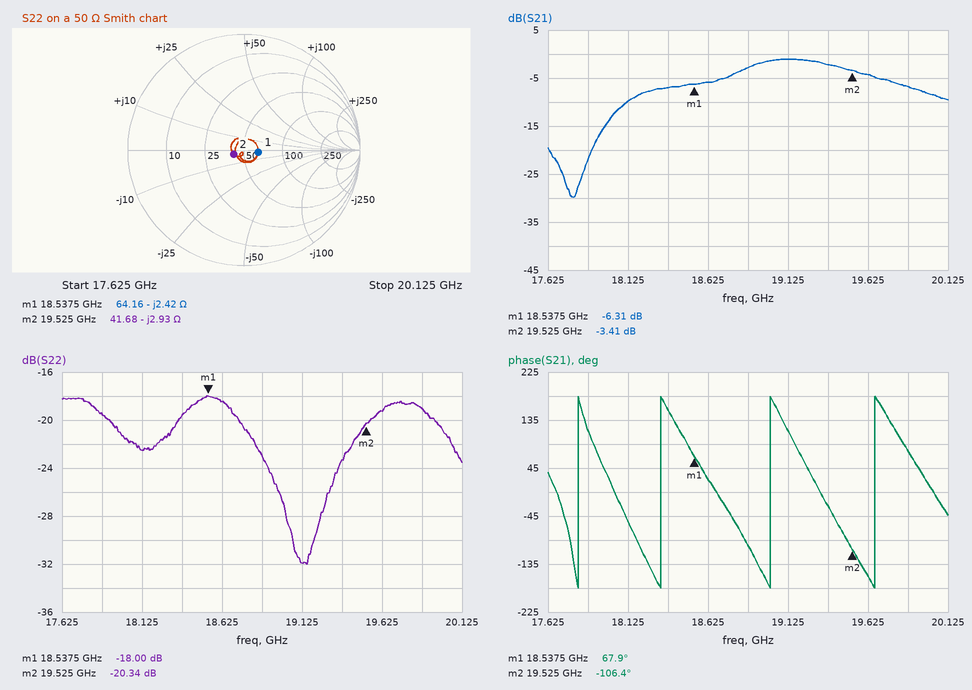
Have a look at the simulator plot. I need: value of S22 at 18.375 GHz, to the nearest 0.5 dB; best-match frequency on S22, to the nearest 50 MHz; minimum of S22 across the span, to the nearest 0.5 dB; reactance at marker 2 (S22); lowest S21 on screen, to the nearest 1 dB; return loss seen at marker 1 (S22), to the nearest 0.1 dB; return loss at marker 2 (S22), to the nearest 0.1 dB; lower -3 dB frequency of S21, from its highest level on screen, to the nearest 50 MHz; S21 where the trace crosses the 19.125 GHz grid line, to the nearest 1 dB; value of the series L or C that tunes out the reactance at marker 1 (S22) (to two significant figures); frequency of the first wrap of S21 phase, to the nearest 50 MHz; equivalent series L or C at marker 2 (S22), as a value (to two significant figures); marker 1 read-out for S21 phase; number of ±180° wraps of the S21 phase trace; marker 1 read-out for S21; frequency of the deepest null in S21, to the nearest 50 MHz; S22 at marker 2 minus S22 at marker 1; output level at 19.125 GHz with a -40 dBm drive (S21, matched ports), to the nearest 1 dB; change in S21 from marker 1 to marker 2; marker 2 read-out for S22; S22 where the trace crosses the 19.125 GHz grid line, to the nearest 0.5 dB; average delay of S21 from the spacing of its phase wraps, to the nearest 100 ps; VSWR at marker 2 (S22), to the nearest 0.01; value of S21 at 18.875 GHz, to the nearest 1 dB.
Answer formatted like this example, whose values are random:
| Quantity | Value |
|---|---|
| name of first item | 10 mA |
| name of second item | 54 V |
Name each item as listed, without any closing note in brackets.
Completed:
| Quantity | Value |
|---|---|
| value of S22 at 18.375 GHz, to the nearest 0.5 dB | -19.5 dB |
| best-match frequency on S22, to the nearest 50 MHz | 19.15 GHz |
| minimum of S22 across the span, to the nearest 0.5 dB | -32.0 dB |
| reactance at marker 2 | -2.93 Ω |
| lowest S21 on screen, to the nearest 1 dB | -30 dB |
| return loss seen at marker 1 (S22), to the nearest 0.1 dB | 18.0 dB |
| return loss at marker 2 (S22), to the nearest 0.1 dB | 20.3 dB |
| lower -3 dB frequency of S21, from its highest level on screen, to the nearest 50 MHz | 18.80 GHz |
| S21 where the trace crosses the 19.125 GHz grid line, to the nearest 1 dB | -1 dB |
| value of the series L or C that tunes out the reactance at marker 1 (S22) | 21 pH |
| frequency of the first wrap of S21 phase, to the nearest 50 MHz | 17.80 GHz |
| equivalent series L or C at marker 2 (S22), as a value | 2.8 pF |
| marker 1 read-out for S21 phase | 67.9° |
| number of ±180° wraps of the S21 phase trace | 4 |
| marker 1 read-out for S21 | -6.31 dB |
| frequency of the deepest null in S21, to the nearest 50 MHz | 17.80 GHz |
| S22 at marker 2 minus S22 at marker 1 | -2.34 dB |
| output level at 19.125 GHz with a -40 dBm drive (S21, matched ports), to the nearest 1 dB | -41 dBm |
| change in S21 from marker 1 to marker 2 | 2.90 dB |
| marker 2 read-out for S22 | -20.34 dB |
| S22 where the trace crosses the 19.125 GHz grid line, to the nearest 0.5 dB | -32.0 dB |
| average delay of S21 from the spacing of its phase wraps, to the nearest 100 ps | 1.6 ns |
| VSWR at marker 2 (S22), to the nearest 0.01 | 1.21 |
| value of S21 at 18.875 GHz, to the nearest 1 dB | -3 dB |
